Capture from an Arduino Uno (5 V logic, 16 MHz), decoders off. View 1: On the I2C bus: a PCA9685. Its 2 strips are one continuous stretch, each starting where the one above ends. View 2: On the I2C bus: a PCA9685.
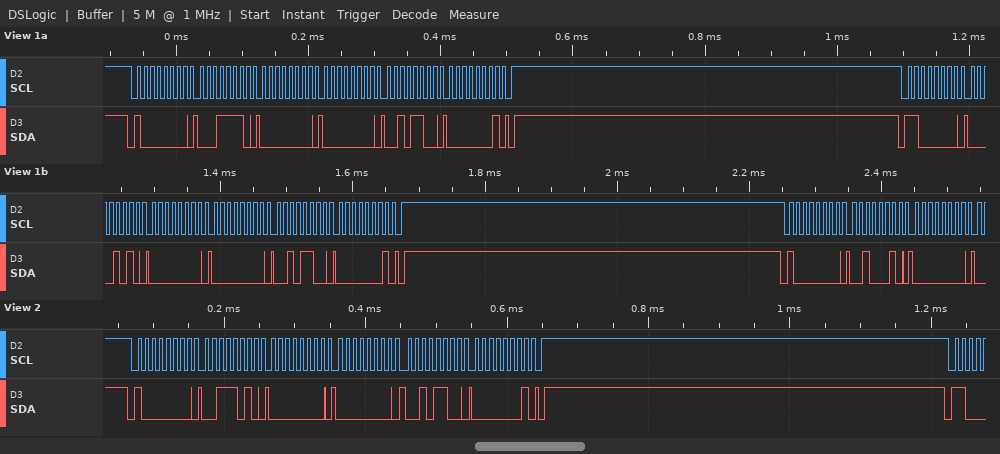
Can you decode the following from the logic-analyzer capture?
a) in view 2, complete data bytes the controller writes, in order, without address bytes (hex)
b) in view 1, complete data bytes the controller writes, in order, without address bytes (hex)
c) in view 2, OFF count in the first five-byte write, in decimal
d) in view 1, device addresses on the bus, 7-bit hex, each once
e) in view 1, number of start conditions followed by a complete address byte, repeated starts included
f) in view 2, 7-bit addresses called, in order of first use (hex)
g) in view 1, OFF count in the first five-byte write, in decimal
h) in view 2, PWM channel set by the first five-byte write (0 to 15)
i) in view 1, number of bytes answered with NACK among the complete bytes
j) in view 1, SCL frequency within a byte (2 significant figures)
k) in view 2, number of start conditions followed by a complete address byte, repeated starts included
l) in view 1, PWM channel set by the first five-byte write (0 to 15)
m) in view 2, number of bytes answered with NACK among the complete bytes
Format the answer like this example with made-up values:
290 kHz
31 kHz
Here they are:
3A 00 00 2C 01
1E 00 00 2C 01 0A 00 00 2C 01 22 00
300
0x40 0x60
3
0x40
300
13
0
100 kHz
1
6
0
